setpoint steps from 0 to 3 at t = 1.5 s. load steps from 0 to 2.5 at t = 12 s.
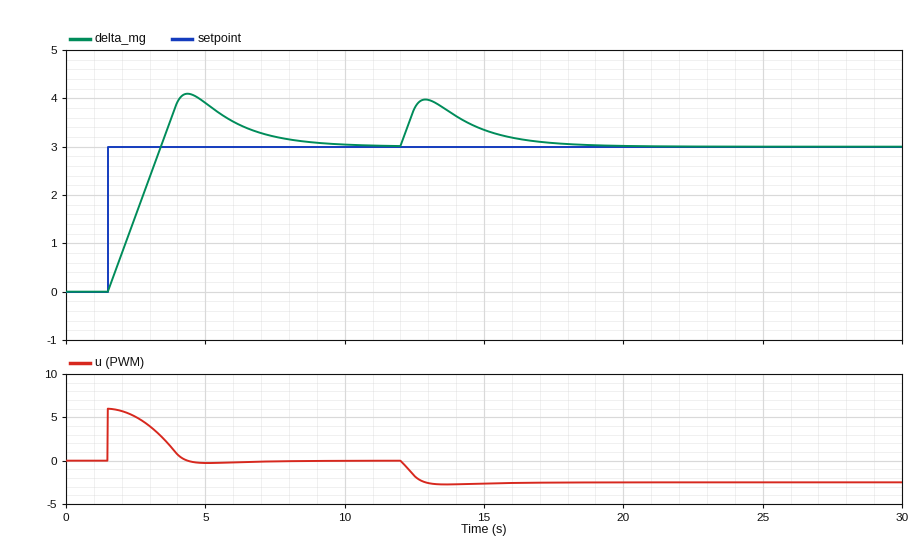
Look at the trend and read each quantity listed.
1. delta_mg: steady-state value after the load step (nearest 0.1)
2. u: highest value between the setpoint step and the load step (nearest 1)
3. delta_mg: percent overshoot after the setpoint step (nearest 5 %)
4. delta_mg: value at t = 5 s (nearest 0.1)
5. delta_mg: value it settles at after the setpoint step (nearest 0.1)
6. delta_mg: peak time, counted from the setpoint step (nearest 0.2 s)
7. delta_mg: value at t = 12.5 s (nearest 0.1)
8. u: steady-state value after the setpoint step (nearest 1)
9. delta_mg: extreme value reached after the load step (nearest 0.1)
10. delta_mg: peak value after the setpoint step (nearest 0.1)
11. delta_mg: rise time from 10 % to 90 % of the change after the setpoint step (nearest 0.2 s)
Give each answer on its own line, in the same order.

3.0
6
35 %
3.9
3.0
2.8 s
3.8
0
4.0
4.1
1.6 s
